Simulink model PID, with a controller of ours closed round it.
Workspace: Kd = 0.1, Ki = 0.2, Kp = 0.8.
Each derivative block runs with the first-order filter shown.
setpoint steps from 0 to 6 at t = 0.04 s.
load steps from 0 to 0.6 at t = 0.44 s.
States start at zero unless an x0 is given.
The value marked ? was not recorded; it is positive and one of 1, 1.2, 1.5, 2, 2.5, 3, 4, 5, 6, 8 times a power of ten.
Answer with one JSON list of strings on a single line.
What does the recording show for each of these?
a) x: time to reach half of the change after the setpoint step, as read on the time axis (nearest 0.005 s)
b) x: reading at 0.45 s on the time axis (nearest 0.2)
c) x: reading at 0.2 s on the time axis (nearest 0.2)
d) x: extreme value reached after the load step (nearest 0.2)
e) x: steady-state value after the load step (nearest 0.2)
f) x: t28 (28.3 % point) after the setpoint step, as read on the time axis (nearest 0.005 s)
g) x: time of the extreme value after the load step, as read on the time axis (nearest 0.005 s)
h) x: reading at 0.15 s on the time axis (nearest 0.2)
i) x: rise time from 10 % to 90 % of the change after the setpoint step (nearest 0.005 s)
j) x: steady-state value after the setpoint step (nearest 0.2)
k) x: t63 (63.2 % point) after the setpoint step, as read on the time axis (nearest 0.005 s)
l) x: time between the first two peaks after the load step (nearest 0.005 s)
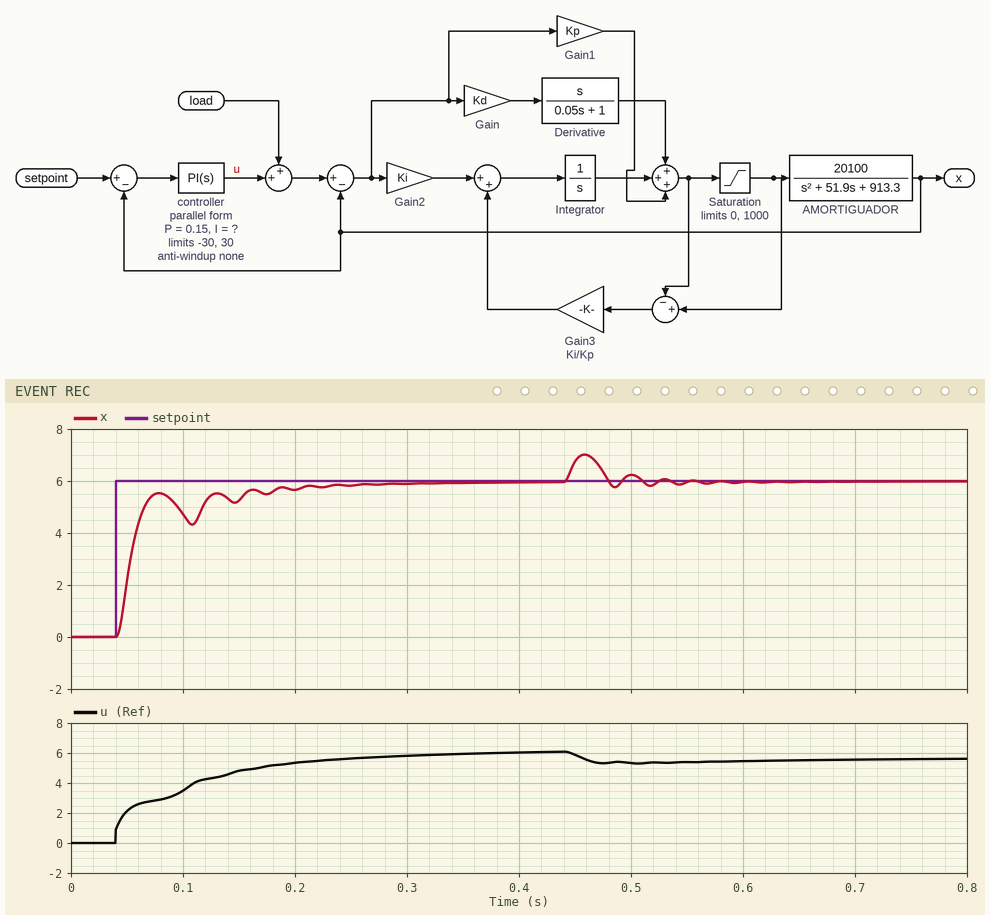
["0.055 s", "6.8", "5.6", "7.0", "6.0", "0.050 s", "0.460 s", "5.2", "0.025 s", "6.0", "0.055 s", "0.040 s"]
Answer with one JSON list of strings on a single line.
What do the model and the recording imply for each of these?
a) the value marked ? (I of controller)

["30"]
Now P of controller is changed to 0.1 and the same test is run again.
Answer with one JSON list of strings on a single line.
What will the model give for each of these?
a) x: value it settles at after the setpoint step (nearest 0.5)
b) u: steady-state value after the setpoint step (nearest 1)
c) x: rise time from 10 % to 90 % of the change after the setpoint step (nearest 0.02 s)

["6.0", "6", "0.08 s"]
